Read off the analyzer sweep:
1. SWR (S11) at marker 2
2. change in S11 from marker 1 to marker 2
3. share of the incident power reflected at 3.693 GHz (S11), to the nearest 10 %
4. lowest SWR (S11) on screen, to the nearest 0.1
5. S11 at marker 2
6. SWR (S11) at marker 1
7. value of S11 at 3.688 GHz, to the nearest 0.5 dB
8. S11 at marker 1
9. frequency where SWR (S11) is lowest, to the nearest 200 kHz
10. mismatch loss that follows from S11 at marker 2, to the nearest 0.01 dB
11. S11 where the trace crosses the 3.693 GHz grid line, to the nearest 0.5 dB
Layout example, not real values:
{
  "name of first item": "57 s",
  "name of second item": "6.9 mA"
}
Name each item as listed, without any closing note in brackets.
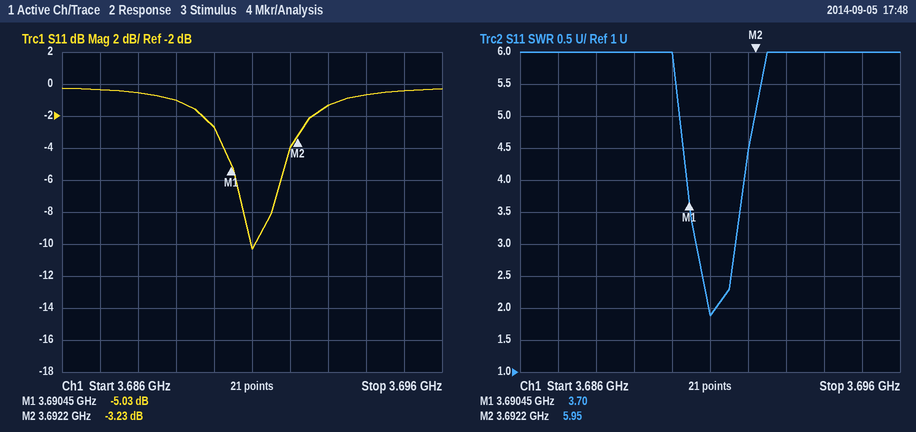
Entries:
{
  "SWR (S11) at marker 2": "5.95",
  "change in S11 from marker 1 to marker 2": "1.80 dB",
  "share of the incident power reflected at 3.693 GHz (S11), to the nearest 10 %": "70 %",
  "lowest SWR (S11) on screen, to the nearest 0.1": "1.9",
  "S11 at marker 2": "-3.23 dB",
  "SWR (S11) at marker 1": "3.70",
  "value of S11 at 3.688 GHz, to the nearest 0.5 dB": "-0.5 dB",
  "S11 at marker 1": "-5.03 dB",
  "frequency where SWR (S11) is lowest, to the nearest 200 kHz": "3.6910 GHz",
  "mismatch loss that follows from S11 at marker 2, to the nearest 0.01 dB": "2.80 dB",
  "S11 where the trace crosses the 3.693 GHz grid line, to the nearest 0.5 dB": "-1.5 dB"
}
